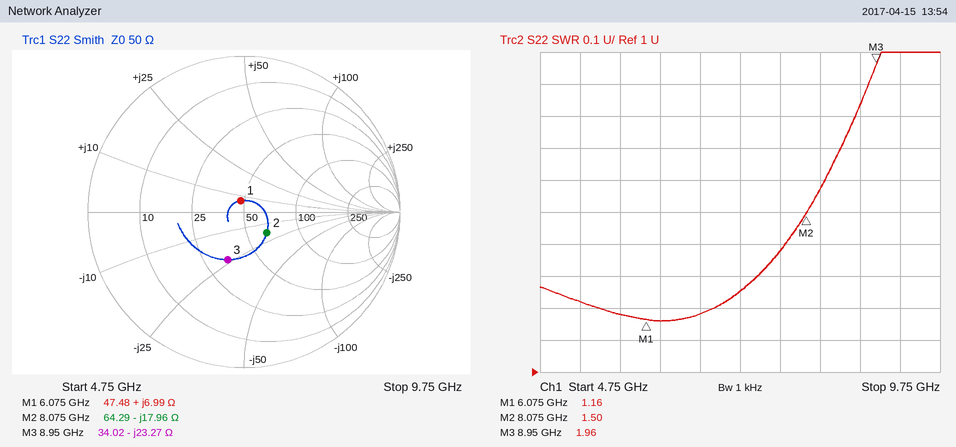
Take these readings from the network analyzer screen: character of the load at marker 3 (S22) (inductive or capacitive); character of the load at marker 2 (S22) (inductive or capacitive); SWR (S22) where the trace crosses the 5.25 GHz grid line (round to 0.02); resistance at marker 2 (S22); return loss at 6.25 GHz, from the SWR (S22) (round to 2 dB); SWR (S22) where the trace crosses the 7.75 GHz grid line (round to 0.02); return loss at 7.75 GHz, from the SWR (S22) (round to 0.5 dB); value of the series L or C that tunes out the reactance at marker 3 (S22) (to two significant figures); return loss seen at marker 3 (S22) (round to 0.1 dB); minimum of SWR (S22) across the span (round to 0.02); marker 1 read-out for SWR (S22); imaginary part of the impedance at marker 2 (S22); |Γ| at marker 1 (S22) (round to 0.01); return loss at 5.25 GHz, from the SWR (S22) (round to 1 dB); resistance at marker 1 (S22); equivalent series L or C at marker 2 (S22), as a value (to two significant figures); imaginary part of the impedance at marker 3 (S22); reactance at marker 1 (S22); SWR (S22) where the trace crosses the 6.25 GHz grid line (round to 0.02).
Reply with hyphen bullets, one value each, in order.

- capacitive
- capacitive
- 1.22
- 64.29 Ω
- 22 dB
- 1.38
- 16.0 dB
- 410 pH
- 9.8 dB
- 1.16
- 1.16
- -17.96 Ω
- 0.08
- 20 dB
- 47.48 Ω
- 1.1 pF
- -23.27 Ω
- +6.99 Ω
- 1.16
